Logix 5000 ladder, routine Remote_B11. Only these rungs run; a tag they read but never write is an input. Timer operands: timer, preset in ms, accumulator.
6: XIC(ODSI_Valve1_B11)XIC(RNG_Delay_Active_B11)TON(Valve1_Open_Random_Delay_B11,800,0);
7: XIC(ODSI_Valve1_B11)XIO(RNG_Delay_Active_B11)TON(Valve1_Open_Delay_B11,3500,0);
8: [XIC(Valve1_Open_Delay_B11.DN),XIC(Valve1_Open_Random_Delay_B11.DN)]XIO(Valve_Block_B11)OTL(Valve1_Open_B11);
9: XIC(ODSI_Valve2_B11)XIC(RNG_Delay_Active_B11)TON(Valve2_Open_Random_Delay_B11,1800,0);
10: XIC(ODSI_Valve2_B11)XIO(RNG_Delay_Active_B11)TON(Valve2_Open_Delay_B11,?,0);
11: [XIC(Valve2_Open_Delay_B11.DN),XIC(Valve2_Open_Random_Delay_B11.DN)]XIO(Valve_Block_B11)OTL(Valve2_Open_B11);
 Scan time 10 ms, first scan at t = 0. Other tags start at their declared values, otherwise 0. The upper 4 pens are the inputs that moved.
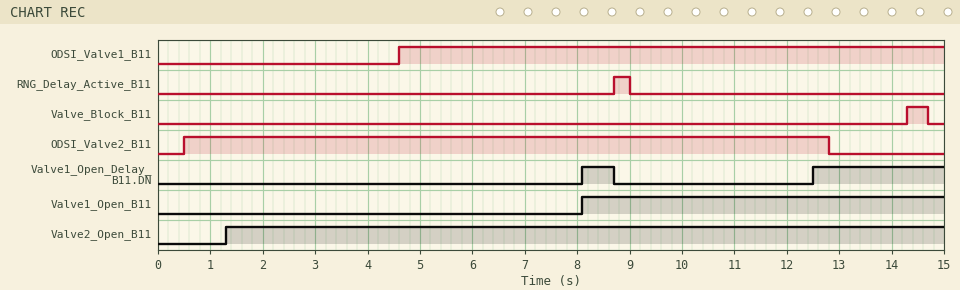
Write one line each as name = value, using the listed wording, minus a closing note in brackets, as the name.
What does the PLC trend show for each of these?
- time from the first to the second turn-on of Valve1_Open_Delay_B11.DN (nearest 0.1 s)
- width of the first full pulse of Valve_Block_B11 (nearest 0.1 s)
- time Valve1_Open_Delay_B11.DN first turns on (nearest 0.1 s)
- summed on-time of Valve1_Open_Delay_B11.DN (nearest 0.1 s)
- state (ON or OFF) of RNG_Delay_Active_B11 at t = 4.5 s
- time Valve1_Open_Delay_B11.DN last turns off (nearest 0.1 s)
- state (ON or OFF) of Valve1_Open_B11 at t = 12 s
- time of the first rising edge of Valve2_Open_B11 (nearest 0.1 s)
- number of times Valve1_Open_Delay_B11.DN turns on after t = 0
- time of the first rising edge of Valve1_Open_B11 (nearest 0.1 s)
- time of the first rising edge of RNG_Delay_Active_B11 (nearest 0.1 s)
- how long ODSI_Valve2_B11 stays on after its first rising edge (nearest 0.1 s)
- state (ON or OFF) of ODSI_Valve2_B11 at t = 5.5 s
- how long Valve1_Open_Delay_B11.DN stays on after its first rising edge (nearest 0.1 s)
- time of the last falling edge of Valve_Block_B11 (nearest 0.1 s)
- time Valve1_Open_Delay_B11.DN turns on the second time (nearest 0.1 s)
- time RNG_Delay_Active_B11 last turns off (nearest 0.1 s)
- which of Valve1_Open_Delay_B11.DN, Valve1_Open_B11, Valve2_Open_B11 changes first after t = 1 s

time from the first to the second turn-on of Valve1_Open_Delay_B11.DN = 4.4 s
width of the first full pulse of Valve_Block_B11 = 0.4 s
time Valve1_Open_Delay_B11.DN first turns on = 8.1 s
summed on-time of Valve1_Open_Delay_B11.DN = 3.1 s
state (ON or OFF) of RNG_Delay_Active_B11 at t = 4.5 s = OFF
time Valve1_Open_Delay_B11.DN last turns off = 8.7 s
state (ON or OFF) of Valve1_Open_B11 at t = 12 s = ON
time of the first rising edge of Valve2_Open_B11 = 1.3 s
number of times Valve1_Open_Delay_B11.DN turns on after t = 0 = 2
time of the first rising edge of Valve1_Open_B11 = 8.1 s
time of the first rising edge of RNG_Delay_Active_B11 = 8.7 s
how long ODSI_Valve2_B11 stays on after its first rising edge = 12.3 s
state (ON or OFF) of ODSI_Valve2_B11 at t = 5.5 s = ON
how long Valve1_Open_Delay_B11.DN stays on after its first rising edge = 0.6 s
time of the last falling edge of Valve_Block_B11 = 14.7 s
time Valve1_Open_Delay_B11.DN turns on the second time = 12.5 s
time RNG_Delay_Active_B11 last turns off = 9.0 s
which of Valve1_Open_Delay_B11.DN, Valve1_Open_B11, Valve2_Open_B11 changes first after t = 1 s = Valve2_Open_B11
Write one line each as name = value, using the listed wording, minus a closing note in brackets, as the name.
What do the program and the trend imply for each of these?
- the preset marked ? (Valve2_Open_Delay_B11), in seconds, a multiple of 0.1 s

the preset marked ? (Valve2_Open_Delay_B11), in seconds, a multiple of 0.1 s = 0.8 s
